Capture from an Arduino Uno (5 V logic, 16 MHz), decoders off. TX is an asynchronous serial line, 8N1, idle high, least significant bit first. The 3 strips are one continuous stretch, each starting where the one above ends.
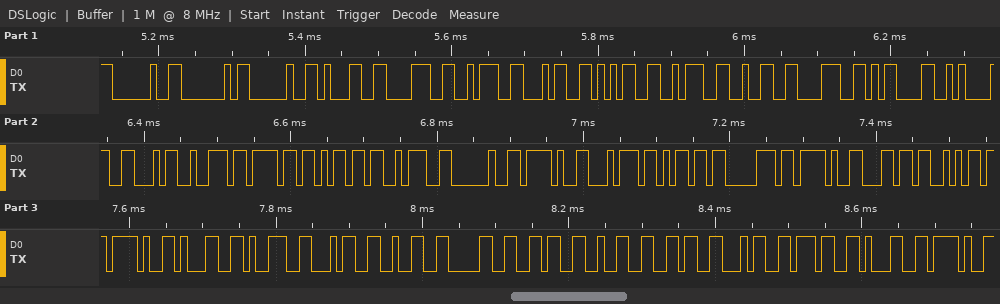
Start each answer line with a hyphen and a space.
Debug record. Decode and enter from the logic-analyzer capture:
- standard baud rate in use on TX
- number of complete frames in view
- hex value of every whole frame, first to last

- 115200 baud
- 39
- 20 40 20 31 38 3A 34 35 3A 32 38 0D 0A 46 72 6F 6D 3A 20 2F 74 6D 70 2F 6C 6A 2F 31 39 34 32 30 36 32 36 34 37 31 2F
